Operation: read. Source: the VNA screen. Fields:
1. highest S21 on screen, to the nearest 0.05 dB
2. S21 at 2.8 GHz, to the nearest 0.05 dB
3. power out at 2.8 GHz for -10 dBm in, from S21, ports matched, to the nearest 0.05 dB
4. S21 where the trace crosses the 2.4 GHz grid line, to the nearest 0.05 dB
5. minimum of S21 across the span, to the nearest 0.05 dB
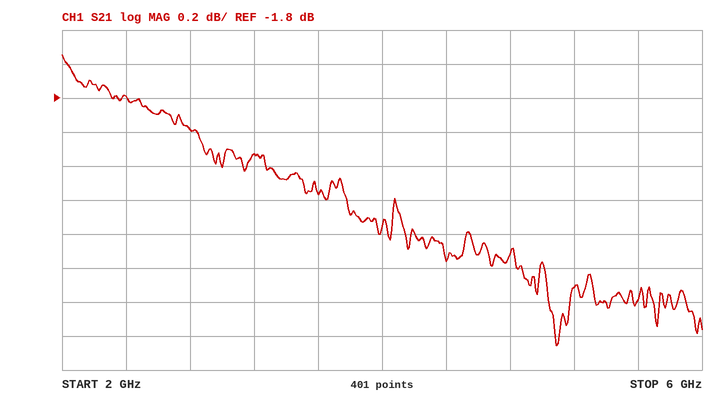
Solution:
-1.55 dB
-2.00 dB
-12.00 dBm
-1.80 dB
-3.25 dB
